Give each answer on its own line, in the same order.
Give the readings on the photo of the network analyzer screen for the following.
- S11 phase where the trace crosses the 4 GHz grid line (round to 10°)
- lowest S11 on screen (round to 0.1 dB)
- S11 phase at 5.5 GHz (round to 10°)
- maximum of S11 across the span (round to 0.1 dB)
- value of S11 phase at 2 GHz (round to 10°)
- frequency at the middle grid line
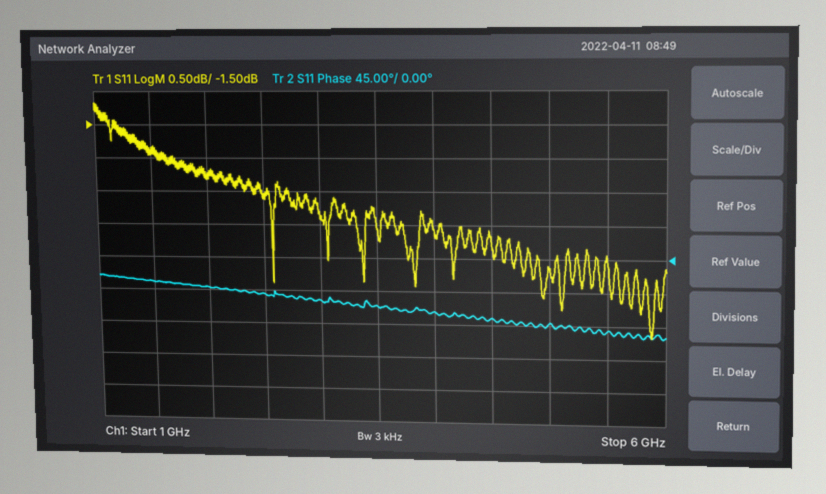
-70°
-4.7 dB
-100°
-1.2 dB
-40°
3.5 GHz
